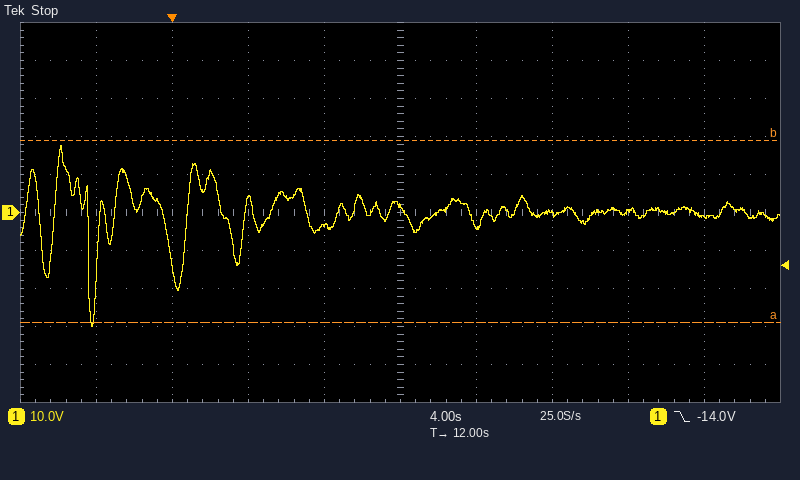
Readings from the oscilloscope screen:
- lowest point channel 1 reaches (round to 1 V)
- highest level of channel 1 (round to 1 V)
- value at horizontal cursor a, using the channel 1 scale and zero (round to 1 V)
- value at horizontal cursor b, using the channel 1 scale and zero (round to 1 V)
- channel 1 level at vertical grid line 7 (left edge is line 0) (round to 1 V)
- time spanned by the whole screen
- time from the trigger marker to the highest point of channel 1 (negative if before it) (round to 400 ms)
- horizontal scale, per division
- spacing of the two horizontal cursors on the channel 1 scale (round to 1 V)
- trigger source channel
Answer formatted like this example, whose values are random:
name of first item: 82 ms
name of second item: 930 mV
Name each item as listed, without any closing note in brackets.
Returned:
lowest point channel 1 reaches: -30 V
highest level of channel 1: 18 V
value at horizontal cursor a, using the channel 1 scale and zero: -29 V
value at horizontal cursor b, using the channel 1 scale and zero: 19 V
channel 1 level at vertical grid line 7 (left edge is line 0): 0 V
time spanned by the whole screen: 40 s
time from the trigger marker to the highest point of channel 1 (negative if before it): -6.0 s
horizontal scale, per division: 4 s
spacing of the two horizontal cursors on the channel 1 scale: 48 V
trigger source channel: channel 1
